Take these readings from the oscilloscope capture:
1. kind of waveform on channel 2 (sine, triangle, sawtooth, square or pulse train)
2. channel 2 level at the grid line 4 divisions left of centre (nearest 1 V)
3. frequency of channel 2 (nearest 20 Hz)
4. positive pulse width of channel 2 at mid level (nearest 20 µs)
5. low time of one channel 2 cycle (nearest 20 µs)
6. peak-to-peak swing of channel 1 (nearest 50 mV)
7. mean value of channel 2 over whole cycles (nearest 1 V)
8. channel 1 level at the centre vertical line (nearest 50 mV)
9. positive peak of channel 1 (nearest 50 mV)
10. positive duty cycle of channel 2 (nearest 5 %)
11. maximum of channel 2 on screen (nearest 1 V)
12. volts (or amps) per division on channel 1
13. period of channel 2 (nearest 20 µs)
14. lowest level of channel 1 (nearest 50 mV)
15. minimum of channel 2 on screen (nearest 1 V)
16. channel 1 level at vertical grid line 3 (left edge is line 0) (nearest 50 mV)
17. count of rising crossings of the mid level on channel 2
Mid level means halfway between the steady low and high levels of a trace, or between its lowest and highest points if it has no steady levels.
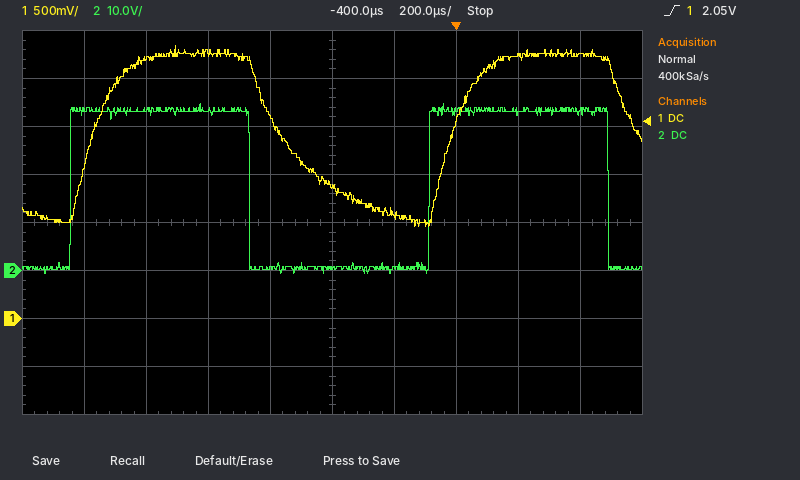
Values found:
square
33 V
860 Hz
580 µs
580 µs
1.90 V
17 V
1.40 V
2.85 V
50 %
35 V
500 mV
1.16 ms
950 mV
-1 V
2.75 V
2
